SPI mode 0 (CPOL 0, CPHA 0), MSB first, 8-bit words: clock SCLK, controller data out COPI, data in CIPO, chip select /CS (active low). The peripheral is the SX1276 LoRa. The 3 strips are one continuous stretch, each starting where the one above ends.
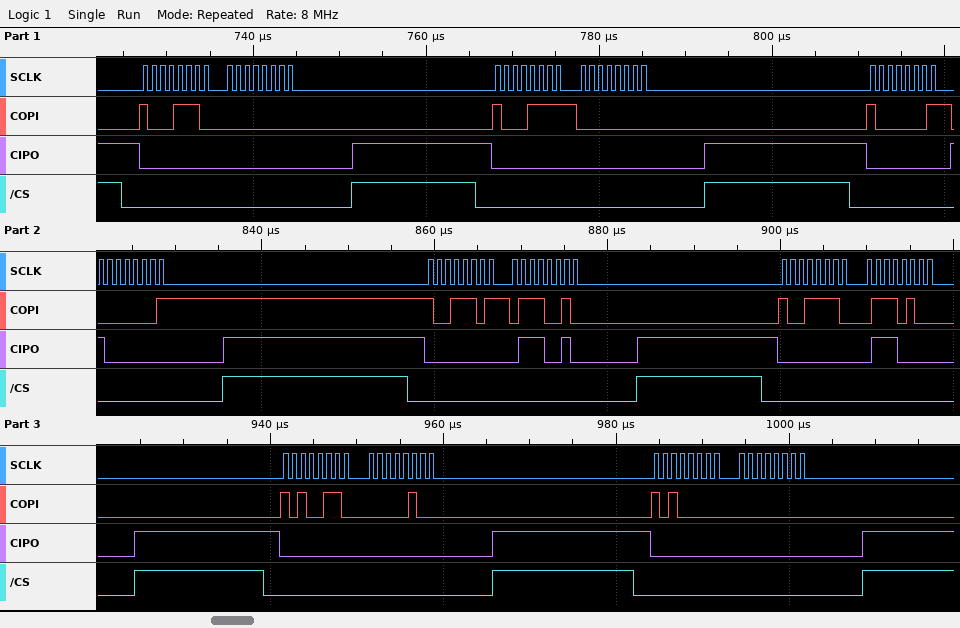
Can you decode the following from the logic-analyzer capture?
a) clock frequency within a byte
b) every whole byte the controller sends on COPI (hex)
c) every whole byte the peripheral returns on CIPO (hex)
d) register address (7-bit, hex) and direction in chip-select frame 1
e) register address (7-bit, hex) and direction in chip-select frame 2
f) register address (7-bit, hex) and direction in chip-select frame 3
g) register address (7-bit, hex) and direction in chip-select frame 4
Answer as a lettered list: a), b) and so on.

a) 1 MHz
b) 8E 00 8F 00 81 01 9D 72 9E 74 A6 04 A0 00
c) 00 00 00 00 00 80 00 72 00 70 00 00 00 00
d) 0x0E write
e) 0x0F write
f) 0x01 write
g) 0x1D write
